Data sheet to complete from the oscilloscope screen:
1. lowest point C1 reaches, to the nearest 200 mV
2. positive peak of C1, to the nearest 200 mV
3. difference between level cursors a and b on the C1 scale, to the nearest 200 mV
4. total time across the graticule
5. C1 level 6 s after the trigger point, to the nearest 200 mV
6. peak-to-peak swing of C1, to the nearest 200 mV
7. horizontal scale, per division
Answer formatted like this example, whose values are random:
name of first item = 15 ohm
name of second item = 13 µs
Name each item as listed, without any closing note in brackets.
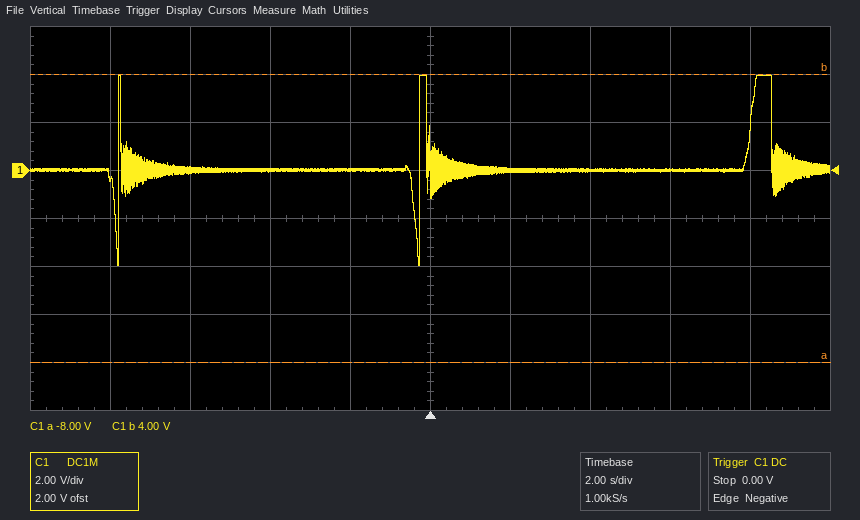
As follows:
lowest point C1 reaches, to the nearest 200 mV = -4.0 V
positive peak of C1, to the nearest 200 mV = 4.0 V
difference between level cursors a and b on the C1 scale, to the nearest 200 mV = 12.0 V
total time across the graticule = 20 s
C1 level 6 s after the trigger point, to the nearest 200 mV = 0.0 V
peak-to-peak swing of C1, to the nearest 200 mV = 8.0 V
horizontal scale, per division = 2 s
